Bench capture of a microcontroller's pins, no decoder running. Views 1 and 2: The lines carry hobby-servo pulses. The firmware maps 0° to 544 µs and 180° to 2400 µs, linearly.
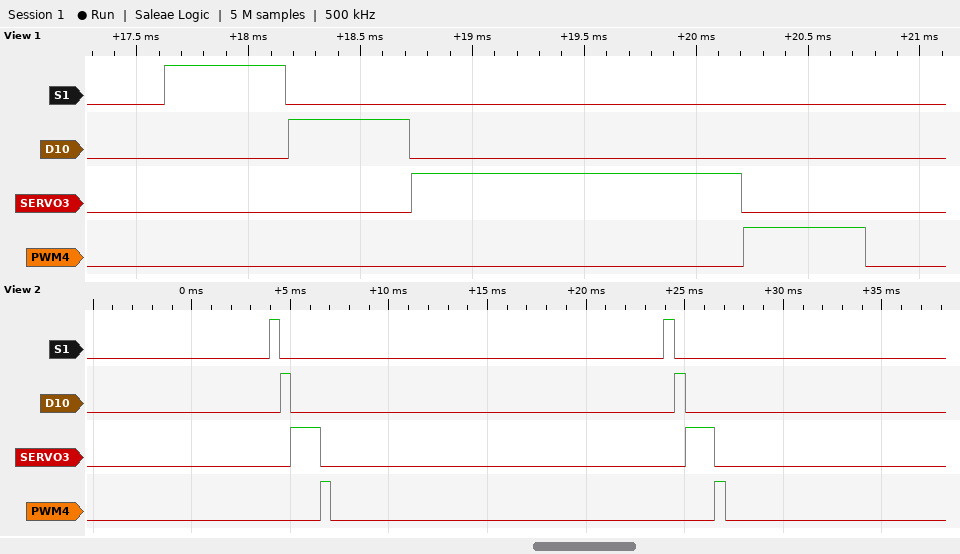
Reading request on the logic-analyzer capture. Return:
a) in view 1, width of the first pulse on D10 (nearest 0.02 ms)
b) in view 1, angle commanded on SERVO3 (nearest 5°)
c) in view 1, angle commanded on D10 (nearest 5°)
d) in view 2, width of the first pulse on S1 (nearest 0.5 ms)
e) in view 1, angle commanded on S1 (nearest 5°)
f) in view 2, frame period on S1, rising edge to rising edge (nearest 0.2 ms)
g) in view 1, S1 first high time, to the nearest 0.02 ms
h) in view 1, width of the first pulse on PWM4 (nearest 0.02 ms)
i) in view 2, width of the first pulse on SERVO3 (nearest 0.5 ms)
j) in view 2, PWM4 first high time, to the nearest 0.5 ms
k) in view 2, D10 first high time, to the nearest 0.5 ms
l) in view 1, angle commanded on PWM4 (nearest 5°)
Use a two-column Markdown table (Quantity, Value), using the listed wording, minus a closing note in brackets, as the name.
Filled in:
| Quantity | Value |
|---|---|
| in view 1, width of the first pulse on D10 | 0.54 ms |
| in view 1, angle commanded on SERVO3 | 90° |
| in view 1, angle commanded on D10 | 0° |
| in view 2, width of the first pulse on S1 | 0.5 ms |
| in view 1, angle commanded on S1 | 0° |
| in view 2, frame period on S1, rising edge to rising edge | 20.0 ms |
| in view 1, S1 first high time, to the nearest 0.02 ms | 0.54 ms |
| in view 1, width of the first pulse on PWM4 | 0.54 ms |
| in view 2, width of the first pulse on SERVO3 | 1.5 ms |
| in view 2, PWM4 first high time, to the nearest 0.5 ms | 0.5 ms |
| in view 2, D10 first high time, to the nearest 0.5 ms | 0.5 ms |
| in view 1, angle commanded on PWM4 | 0° |
